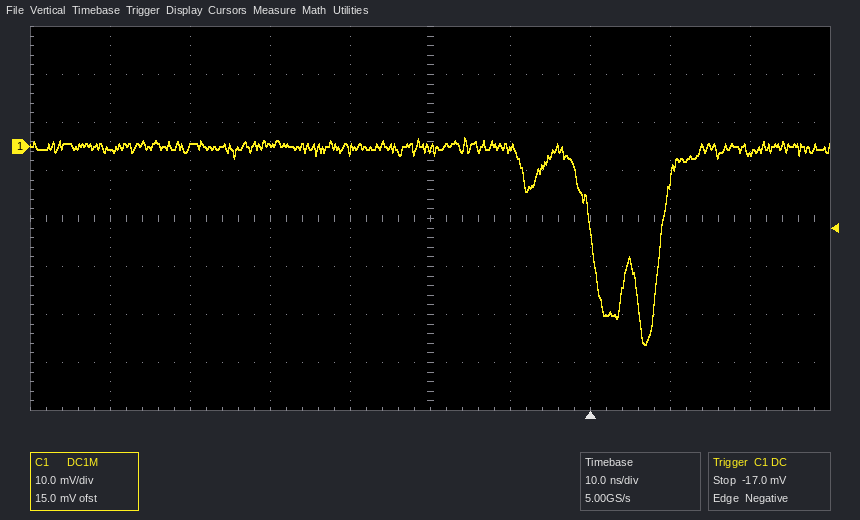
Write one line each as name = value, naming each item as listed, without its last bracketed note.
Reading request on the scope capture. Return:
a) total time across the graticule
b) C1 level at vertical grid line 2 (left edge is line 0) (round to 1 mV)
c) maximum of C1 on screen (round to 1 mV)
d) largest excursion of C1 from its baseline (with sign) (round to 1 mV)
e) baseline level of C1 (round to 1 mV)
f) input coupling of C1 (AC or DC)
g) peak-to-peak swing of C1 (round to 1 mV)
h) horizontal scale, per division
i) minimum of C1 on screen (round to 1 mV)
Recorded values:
total time across the graticule = 100 ns
C1 level at vertical grid line 2 (left edge is line 0) = 0 mV
maximum of C1 on screen = 2 mV
largest excursion of C1 from its baseline (with sign) = -41 mV
baseline level of C1 = 0 mV
input coupling of C1 = DC
peak-to-peak swing of C1 = 43 mV
horizontal scale, per division = 10 ns
minimum of C1 on screen = -41 mV
